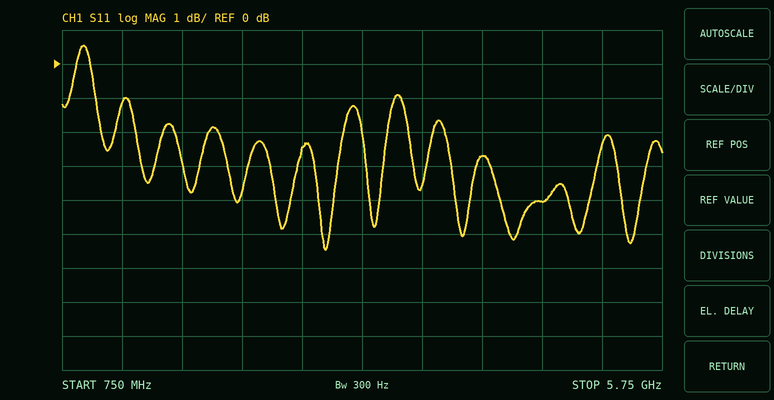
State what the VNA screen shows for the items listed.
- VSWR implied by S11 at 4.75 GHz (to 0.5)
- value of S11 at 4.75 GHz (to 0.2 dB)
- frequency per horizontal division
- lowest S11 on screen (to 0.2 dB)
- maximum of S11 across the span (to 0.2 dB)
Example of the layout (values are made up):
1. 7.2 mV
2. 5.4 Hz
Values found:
1. 4.5
2. -4.0 dB
3. 500 MHz
4. -5.4 dB
5. 0.6 dB
